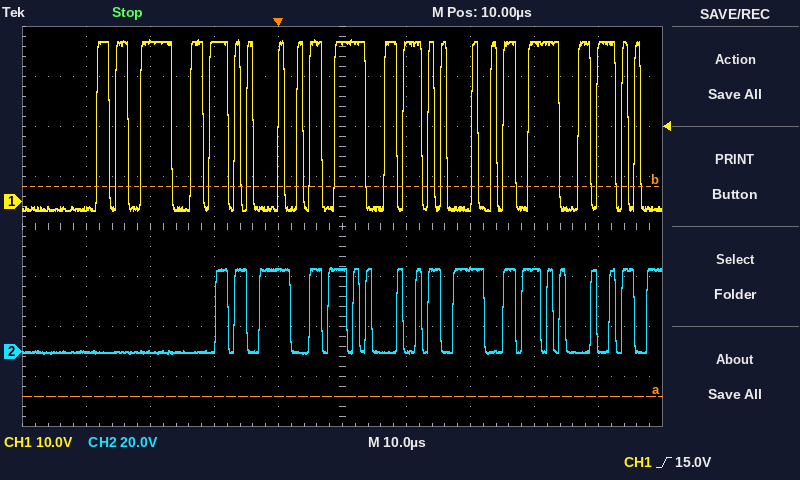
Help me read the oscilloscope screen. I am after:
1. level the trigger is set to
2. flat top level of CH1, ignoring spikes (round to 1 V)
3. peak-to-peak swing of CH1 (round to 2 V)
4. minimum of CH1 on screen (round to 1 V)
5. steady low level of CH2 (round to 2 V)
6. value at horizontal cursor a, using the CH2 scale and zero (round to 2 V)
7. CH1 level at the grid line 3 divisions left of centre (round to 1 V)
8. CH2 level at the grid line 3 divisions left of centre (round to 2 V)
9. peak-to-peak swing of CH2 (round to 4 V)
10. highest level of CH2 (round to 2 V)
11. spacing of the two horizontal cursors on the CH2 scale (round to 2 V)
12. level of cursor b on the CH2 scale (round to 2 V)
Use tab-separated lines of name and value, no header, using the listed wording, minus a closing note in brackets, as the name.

level the trigger is set to	15.0 V
flat top level of CH1, ignoring spikes	32 V
peak-to-peak swing of CH1	34 V
minimum of CH1 on screen	-2 V
steady low level of CH2	0 V
value at horizontal cursor a, using the CH2 scale and zero	-18 V
CH1 level at the grid line 3 divisions left of centre	32 V
CH2 level at the grid line 3 divisions left of centre	0 V
peak-to-peak swing of CH2	36 V
highest level of CH2	34 V
spacing of the two horizontal cursors on the CH2 scale	84 V
level of cursor b on the CH2 scale	66 V
